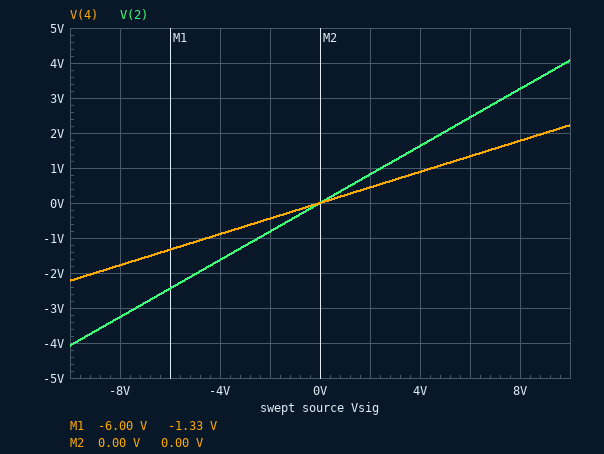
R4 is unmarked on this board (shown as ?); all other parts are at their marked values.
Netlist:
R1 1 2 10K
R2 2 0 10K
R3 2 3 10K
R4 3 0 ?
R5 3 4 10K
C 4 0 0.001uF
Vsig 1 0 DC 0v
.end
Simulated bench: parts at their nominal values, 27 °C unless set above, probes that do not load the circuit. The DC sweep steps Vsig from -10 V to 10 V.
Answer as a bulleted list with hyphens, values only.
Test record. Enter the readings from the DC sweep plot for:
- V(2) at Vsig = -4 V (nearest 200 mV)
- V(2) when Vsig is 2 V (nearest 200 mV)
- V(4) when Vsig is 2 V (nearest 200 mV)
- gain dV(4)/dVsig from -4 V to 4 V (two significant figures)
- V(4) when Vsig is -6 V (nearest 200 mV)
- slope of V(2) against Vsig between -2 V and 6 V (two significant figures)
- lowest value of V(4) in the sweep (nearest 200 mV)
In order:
- -1.6 V
- 800 mV
- 400 mV
- 0.22 V/V
- -1.4 V
- 0.41 V/V
- -2.2 V
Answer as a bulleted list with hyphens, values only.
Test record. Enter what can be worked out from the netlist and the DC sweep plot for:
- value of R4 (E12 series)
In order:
- 12 kΩ
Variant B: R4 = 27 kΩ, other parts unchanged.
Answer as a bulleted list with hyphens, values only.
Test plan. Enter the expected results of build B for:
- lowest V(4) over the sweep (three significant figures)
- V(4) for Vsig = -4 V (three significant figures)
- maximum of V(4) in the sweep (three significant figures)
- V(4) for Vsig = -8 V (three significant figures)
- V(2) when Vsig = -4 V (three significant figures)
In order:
- -3.21 V
- -1.29 V
- 3.21 V
- -2.57 V
- -1.76 V
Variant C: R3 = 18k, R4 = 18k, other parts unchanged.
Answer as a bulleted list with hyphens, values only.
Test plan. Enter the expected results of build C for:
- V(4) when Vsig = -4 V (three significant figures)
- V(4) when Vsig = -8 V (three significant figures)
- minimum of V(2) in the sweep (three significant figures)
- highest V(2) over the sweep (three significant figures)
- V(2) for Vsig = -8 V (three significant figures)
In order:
- -878 mV
- -1.76 V
- -4.39 V
- 4.39 V
- -3.51 V
